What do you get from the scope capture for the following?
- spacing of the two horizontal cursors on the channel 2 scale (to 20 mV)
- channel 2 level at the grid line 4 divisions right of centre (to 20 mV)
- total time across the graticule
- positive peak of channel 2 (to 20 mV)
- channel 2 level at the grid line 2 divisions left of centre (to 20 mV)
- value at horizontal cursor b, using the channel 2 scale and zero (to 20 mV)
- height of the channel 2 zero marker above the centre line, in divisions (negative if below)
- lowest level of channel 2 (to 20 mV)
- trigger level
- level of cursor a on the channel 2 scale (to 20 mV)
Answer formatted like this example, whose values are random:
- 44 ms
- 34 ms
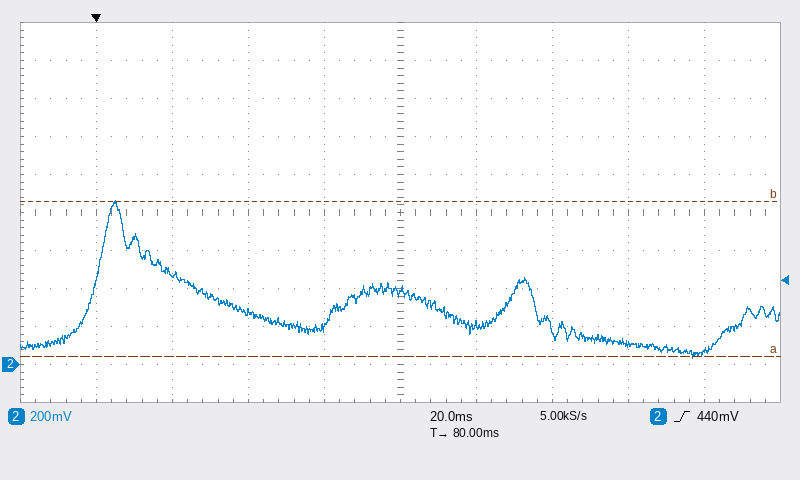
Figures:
- 820 mV
- 60 mV
- 200 ms
- 860 mV
- 280 mV
- 860 mV
- -4.0 div
- 40 mV
- 440 mV
- 40 mV
